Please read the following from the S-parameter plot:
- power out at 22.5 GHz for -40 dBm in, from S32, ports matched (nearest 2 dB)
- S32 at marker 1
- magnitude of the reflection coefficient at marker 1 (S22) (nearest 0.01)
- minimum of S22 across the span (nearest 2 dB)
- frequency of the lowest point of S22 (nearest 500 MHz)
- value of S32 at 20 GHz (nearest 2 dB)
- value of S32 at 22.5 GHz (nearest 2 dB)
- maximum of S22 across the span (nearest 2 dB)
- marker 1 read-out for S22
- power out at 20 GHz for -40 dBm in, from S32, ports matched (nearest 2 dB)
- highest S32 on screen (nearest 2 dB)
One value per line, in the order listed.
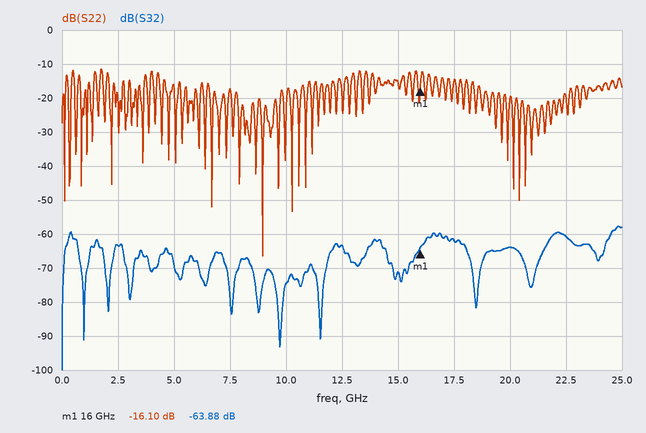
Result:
-100 dBm
-63.88 dB
0.16
-66 dB
9.0 GHz
-64 dB
-60 dB
-12 dB
-16.10 dB
-104 dBm
-58 dB
